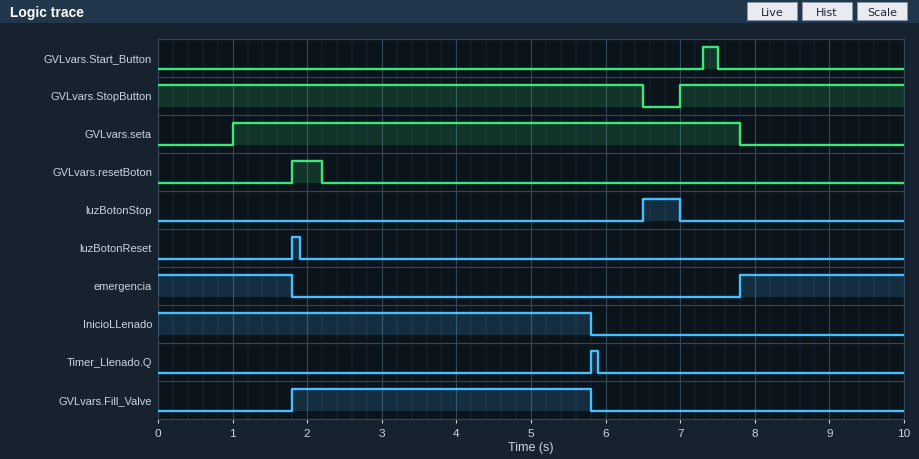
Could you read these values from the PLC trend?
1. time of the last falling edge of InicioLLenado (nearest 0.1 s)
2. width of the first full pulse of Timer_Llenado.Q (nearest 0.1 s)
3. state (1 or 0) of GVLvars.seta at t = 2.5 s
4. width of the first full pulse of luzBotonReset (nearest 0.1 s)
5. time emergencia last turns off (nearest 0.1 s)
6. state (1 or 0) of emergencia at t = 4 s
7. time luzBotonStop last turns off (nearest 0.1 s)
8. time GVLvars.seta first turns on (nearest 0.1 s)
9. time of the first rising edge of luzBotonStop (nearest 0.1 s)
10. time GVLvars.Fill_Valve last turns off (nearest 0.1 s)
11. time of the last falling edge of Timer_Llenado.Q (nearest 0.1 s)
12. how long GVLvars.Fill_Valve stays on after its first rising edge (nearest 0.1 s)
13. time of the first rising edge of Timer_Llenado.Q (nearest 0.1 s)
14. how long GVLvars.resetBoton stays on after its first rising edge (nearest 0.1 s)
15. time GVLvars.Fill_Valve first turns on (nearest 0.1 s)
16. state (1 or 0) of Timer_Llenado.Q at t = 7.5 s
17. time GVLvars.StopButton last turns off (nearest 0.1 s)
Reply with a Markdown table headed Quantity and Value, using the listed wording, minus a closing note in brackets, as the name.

| Quantity | Value |
|---|---|
| time of the last falling edge of InicioLLenado | 5.8 s |
| width of the first full pulse of Timer_Llenado.Q | 0.1 s |
| state (1 or 0) of GVLvars.seta at t = 2.5 s | 1 |
| width of the first full pulse of luzBotonReset | 0.1 s |
| time emergencia last turns off | 1.8 s |
| state (1 or 0) of emergencia at t = 4 s | 0 |
| time luzBotonStop last turns off | 7.0 s |
| time GVLvars.seta first turns on | 1.0 s |
| time of the first rising edge of luzBotonStop | 6.5 s |
| time GVLvars.Fill_Valve last turns off | 5.8 s |
| time of the last falling edge of Timer_Llenado.Q | 5.9 s |
| how long GVLvars.Fill_Valve stays on after its first rising edge | 4.0 s |
| time of the first rising edge of Timer_Llenado.Q | 5.8 s |
| how long GVLvars.resetBoton stays on after its first rising edge | 0.4 s |
| time GVLvars.Fill_Valve first turns on | 1.8 s |
| state (1 or 0) of Timer_Llenado.Q at t = 7.5 s | 0 |
| time GVLvars.StopButton last turns off | 6.5 s |
